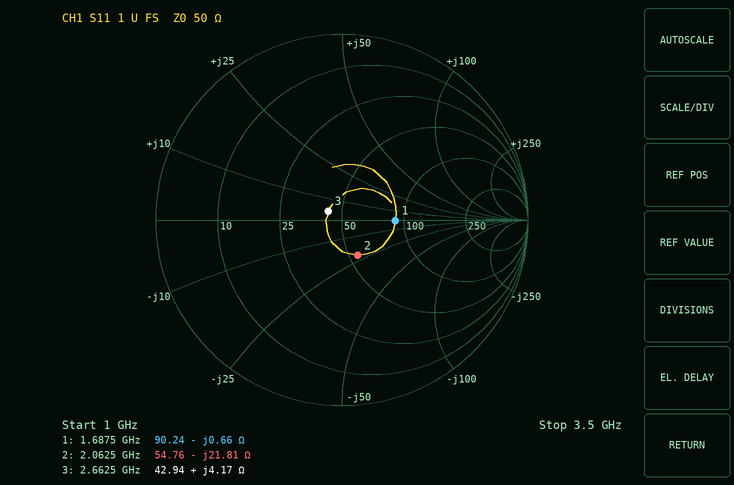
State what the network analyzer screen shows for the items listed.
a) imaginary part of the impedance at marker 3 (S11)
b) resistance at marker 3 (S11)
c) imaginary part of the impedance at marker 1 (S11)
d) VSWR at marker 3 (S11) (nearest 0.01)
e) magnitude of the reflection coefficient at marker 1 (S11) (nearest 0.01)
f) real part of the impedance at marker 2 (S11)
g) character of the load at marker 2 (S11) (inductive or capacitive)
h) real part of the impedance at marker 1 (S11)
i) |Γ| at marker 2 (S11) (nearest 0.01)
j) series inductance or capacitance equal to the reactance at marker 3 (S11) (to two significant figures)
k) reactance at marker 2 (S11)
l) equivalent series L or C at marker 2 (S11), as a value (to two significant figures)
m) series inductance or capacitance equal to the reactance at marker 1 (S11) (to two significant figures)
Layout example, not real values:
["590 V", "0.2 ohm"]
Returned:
["+4.17 Ω", "42.94 Ω", "-0.66 Ω", "1.19", "0.29", "54.76 Ω", "capacitive", "90.24 Ω", "0.21", "250 pH", "-21.81 Ω", "3.5 pF", "140 pF"]
